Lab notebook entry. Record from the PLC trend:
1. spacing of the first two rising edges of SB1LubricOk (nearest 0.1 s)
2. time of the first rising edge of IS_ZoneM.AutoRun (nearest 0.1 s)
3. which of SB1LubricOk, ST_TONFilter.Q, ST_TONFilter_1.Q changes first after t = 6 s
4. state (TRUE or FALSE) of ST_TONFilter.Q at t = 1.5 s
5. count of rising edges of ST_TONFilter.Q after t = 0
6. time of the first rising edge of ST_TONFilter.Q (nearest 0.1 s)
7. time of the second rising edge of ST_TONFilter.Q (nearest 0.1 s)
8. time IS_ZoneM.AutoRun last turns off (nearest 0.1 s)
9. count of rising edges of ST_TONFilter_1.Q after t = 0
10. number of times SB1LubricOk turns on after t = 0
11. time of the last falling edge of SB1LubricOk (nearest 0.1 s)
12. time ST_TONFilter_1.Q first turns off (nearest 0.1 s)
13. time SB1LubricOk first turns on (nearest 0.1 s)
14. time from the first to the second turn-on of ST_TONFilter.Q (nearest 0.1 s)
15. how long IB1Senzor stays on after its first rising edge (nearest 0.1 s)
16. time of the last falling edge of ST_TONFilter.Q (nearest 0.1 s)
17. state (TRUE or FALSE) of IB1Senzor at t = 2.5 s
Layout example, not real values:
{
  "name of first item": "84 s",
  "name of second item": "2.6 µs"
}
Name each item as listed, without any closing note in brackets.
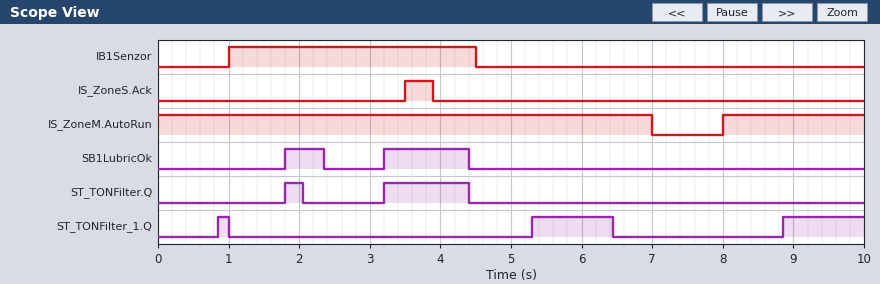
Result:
{
  "spacing of the first two rising edges of SB1LubricOk": "1.4 s",
  "time of the first rising edge of IS_ZoneM.AutoRun": "8.0 s",
  "which of SB1LubricOk, ST_TONFilter.Q, ST_TONFilter_1.Q changes first after t = 6 s": "ST_TONFilter_1.Q",
  "state (TRUE or FALSE) of ST_TONFilter.Q at t = 1.5 s": "FALSE",
  "count of rising edges of ST_TONFilter.Q after t = 0": "2",
  "time of the first rising edge of ST_TONFilter.Q": "1.8 s",
  "time of the second rising edge of ST_TONFilter.Q": "3.2 s",
  "time IS_ZoneM.AutoRun last turns off": "7.0 s",
  "count of rising edges of ST_TONFilter_1.Q after t = 0": "3",
  "number of times SB1LubricOk turns on after t = 0": "2",
  "time of the last falling edge of SB1LubricOk": "4.4 s",
  "time ST_TONFilter_1.Q first turns off": "1.0 s",
  "time SB1LubricOk first turns on": "1.8 s",
  "time from the first to the second turn-on of ST_TONFilter.Q": "1.4 s",
  "how long IB1Senzor stays on after its first rising edge": "3.5 s",
  "time of the last falling edge of ST_TONFilter.Q": "4.4 s",
  "state (TRUE or FALSE) of IB1Senzor at t = 2.5 s": "TRUE"
}
